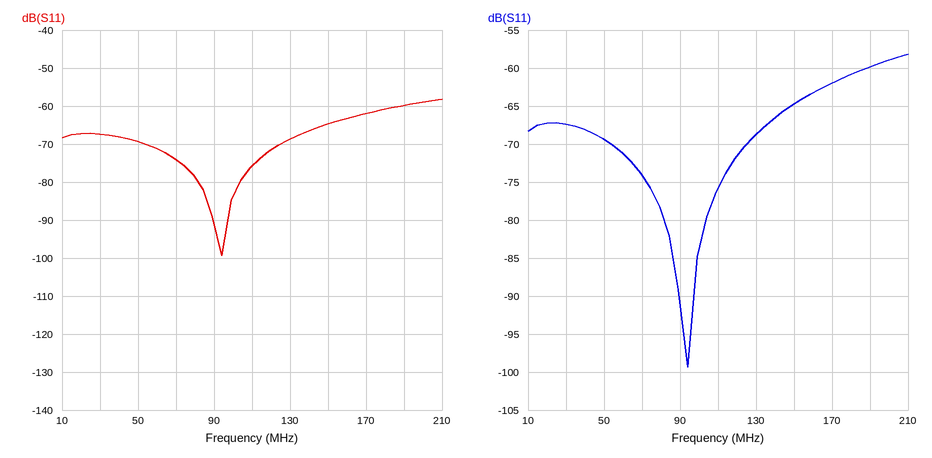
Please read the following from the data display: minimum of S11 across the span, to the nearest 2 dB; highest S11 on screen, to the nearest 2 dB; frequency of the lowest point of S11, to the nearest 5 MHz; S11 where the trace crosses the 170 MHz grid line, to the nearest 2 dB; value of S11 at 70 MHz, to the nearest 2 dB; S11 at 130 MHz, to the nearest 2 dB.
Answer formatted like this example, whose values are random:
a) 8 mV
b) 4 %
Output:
a) -100 dB
b) -58 dB
c) 95 MHz
d) -62 dB
e) -74 dB
f) -68 dB
